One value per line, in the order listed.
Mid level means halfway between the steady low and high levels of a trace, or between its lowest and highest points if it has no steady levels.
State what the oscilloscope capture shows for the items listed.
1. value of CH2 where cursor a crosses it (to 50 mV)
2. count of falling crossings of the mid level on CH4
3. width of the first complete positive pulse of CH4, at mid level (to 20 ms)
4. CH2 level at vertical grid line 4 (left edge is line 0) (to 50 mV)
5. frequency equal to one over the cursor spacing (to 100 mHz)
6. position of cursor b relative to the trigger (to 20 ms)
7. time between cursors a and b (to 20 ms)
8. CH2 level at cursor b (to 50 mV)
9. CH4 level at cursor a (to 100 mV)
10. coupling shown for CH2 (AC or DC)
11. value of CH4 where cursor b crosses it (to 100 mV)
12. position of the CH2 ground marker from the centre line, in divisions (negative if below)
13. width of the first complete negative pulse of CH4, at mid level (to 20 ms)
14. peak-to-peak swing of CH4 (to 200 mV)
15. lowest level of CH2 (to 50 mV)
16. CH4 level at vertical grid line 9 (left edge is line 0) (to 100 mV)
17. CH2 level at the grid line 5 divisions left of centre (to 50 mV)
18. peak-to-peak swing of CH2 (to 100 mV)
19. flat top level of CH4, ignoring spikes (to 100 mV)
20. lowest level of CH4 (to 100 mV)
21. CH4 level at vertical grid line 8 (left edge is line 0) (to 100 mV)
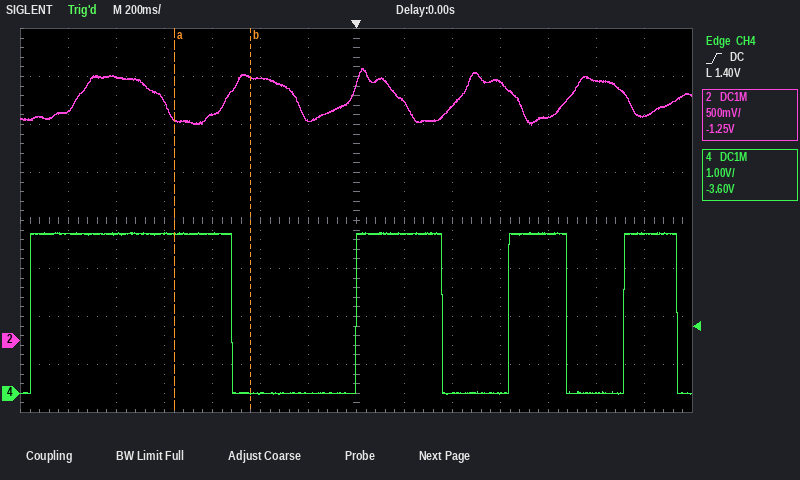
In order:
2.30 V
4
840 ms
2.35 V
3.1 Hz
-440 ms
320 ms
2.75 V
3.3 V
DC
0.0 V
-2.5 div
520 ms
3.4 V
2.25 V
0.0 V
2.75 V
600 mV
3.3 V
0.0 V
3.3 V
